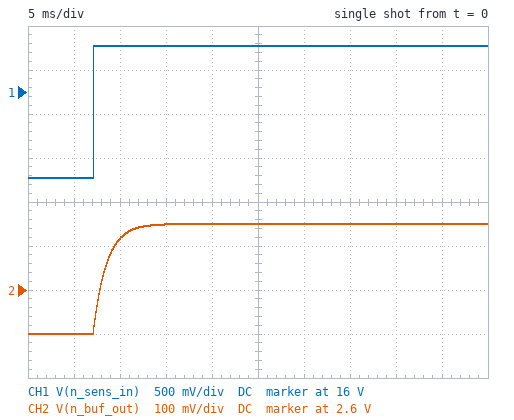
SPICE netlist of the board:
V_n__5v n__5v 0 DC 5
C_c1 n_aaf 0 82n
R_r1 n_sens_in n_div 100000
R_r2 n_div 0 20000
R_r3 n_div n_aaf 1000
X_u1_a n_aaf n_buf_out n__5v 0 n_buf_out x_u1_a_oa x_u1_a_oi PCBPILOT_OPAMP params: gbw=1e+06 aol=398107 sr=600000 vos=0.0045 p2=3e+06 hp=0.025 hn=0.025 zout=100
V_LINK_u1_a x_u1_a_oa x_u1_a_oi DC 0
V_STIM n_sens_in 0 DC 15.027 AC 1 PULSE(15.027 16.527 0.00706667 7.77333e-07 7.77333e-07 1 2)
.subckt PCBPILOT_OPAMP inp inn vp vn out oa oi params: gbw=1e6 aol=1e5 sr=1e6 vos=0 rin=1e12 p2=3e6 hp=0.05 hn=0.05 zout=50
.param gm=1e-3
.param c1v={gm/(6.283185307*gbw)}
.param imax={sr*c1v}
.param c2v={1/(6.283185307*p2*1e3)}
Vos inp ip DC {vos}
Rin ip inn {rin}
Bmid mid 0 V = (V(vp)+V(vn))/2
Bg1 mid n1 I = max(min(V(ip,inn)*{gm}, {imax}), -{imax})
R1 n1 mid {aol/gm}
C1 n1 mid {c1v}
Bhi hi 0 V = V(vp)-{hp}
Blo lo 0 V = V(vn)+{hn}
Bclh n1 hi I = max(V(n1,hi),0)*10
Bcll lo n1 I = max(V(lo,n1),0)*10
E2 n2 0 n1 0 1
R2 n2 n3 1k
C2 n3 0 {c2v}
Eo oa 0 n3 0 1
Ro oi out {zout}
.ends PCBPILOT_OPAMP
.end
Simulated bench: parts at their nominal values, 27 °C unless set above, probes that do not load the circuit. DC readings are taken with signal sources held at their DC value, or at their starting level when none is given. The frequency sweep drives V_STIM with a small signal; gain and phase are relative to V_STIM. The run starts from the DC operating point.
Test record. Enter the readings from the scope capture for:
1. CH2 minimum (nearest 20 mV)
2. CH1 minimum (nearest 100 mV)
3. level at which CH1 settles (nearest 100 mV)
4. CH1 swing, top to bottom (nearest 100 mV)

2.50 V
15.0 V
16.5 V
1.5 V
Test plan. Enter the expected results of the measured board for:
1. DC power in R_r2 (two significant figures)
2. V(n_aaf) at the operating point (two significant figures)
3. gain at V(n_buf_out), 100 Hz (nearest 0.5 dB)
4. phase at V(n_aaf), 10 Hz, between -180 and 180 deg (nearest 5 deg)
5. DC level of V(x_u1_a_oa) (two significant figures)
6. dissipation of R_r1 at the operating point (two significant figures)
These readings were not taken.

310 µW
2.5 V
-18.0 dB
-5 deg
2.5 V
1.6 mW
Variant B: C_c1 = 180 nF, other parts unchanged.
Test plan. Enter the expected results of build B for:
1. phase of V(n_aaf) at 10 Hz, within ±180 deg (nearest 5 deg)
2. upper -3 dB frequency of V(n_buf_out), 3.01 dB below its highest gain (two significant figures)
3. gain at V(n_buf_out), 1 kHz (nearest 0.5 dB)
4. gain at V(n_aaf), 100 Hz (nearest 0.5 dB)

-10 deg
50 Hz
-41.5 dB
-22.5 dB
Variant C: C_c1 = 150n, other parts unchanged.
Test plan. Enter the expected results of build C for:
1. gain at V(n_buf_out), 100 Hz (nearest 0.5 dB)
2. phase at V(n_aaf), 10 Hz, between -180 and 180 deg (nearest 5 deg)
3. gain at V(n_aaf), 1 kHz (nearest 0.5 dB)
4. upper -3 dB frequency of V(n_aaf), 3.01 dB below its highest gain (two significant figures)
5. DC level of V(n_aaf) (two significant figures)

-21.5 dB
-10 deg
-40.0 dB
60 Hz
2.5 V
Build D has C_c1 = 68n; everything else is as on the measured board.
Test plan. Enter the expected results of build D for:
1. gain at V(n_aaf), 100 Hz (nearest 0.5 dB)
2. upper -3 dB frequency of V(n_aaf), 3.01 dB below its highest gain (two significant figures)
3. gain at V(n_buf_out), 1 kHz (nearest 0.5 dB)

-17.5 dB
130 Hz
-33.0 dB
